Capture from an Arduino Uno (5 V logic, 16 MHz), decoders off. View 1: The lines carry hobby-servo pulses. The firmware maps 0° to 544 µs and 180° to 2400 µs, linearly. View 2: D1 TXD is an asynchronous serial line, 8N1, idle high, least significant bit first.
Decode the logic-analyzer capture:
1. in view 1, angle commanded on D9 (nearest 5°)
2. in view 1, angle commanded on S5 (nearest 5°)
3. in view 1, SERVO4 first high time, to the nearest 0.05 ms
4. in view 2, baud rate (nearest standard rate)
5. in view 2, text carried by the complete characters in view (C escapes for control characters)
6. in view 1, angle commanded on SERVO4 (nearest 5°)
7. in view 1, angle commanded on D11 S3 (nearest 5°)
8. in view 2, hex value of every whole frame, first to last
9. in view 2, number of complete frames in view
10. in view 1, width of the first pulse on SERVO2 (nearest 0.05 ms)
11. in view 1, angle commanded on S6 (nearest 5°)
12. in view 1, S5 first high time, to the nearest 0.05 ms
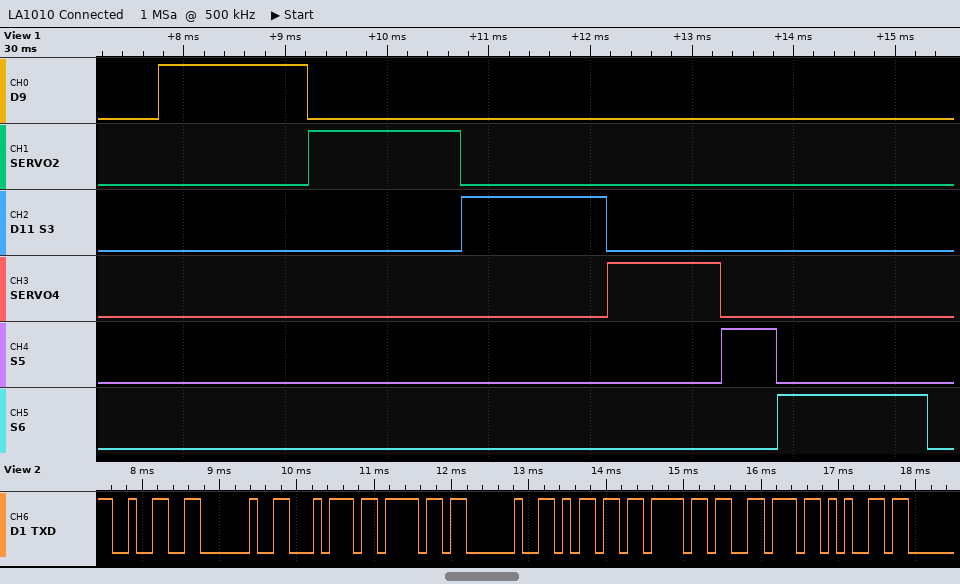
90°
0°
1.10 ms
9600 baud
"2 to move"
55°
85°
32 20 74 6F 20 6D 6F 76 65
9
1.50 ms
90°
0.55 ms
